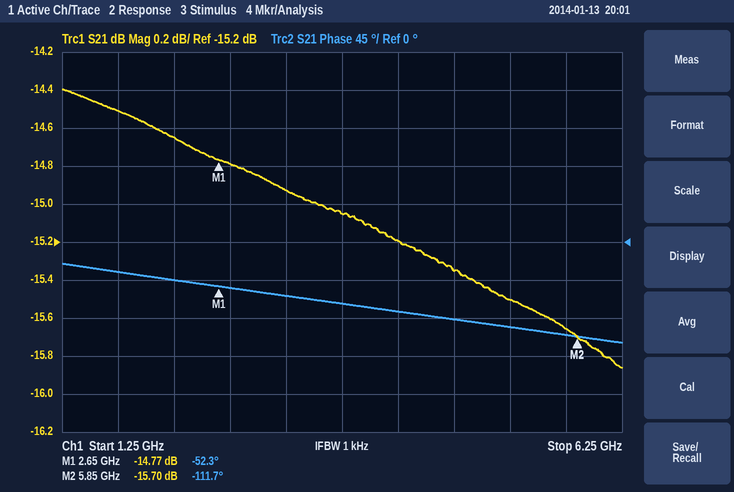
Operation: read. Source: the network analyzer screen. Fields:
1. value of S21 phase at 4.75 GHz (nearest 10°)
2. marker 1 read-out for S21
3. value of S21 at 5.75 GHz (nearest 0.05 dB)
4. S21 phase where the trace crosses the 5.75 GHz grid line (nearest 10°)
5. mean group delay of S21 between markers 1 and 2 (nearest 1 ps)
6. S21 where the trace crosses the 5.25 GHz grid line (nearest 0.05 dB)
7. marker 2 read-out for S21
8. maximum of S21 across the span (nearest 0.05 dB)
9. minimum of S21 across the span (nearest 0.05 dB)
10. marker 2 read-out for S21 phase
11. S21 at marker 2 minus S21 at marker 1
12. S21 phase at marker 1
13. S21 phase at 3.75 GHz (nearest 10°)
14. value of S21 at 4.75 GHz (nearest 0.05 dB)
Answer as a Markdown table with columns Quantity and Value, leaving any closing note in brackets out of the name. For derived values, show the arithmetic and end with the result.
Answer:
| Quantity | Value |
|---|---|
| value of S21 phase at 4.75 GHz | -90° |
| marker 1 read-out for S21 | -14.77 dB |
| value of S21 at 5.75 GHz | -15.65 dB |
| S21 phase where the trace crosses the 5.75 GHz grid line | -110° |
| mean group delay of S21 between markers 1 and 2 | −(-111.7° − (-52.3°))/(360° × 3.2 GHz) ≈ 52 ps |
| S21 where the trace crosses the 5.25 GHz grid line | -15.50 dB |
| marker 2 read-out for S21 | -15.70 dB |
| maximum of S21 across the span | -14.40 dB |
| minimum of S21 across the span | -15.85 dB |
| marker 2 read-out for S21 phase | -111.7° |
| S21 at marker 2 minus S21 at marker 1 | -15.7 − (-14.77) = -0.93 dB |
| S21 phase at marker 1 | -52.3° |
| S21 phase at 3.75 GHz | -70° |
| value of S21 at 4.75 GHz | -15.35 dB |
